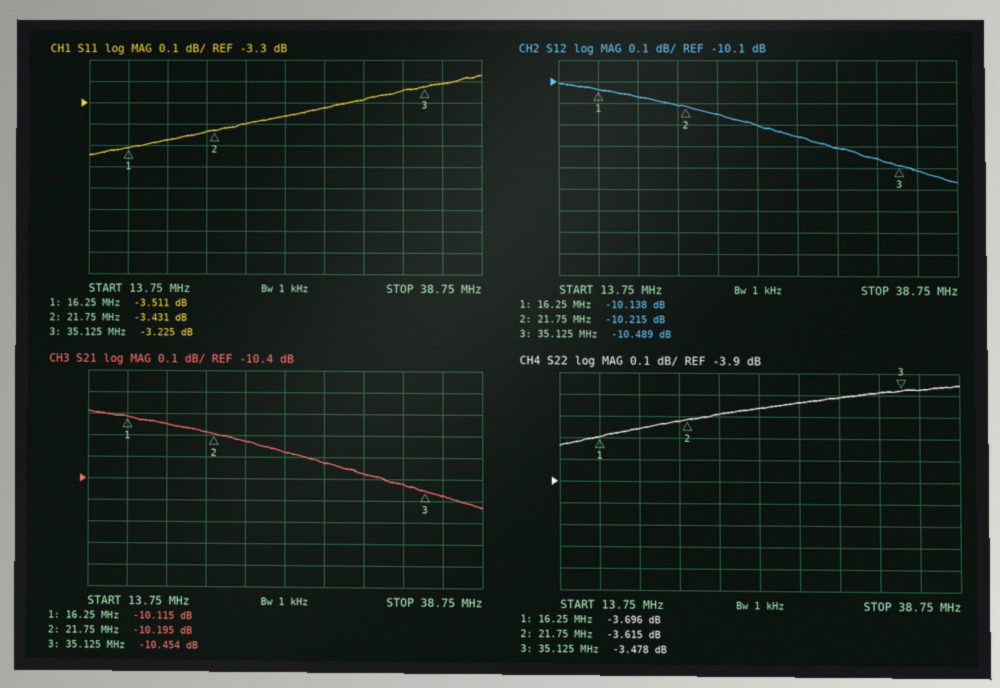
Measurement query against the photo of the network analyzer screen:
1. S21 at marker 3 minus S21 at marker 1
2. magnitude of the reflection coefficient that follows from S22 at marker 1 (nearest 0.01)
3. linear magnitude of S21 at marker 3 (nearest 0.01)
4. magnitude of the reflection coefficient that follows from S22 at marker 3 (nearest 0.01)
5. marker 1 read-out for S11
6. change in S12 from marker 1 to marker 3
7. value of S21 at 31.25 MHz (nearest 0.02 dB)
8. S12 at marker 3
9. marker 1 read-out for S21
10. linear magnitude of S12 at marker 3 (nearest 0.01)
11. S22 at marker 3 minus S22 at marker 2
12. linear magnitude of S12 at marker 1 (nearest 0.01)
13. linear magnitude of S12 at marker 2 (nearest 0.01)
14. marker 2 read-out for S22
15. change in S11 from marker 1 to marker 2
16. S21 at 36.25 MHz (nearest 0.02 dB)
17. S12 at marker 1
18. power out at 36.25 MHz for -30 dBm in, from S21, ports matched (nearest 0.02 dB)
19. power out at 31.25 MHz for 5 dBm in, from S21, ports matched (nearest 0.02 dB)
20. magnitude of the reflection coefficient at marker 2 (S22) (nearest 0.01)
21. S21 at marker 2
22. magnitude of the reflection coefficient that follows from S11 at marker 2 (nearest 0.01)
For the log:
-0.339 dB
0.65
0.30
0.67
-3.511 dB
-0.351 dB
-10.38 dB
-10.489 dB
-10.115 dB
0.30
0.137 dB
0.31
0.31
-3.615 dB
0.080 dB
-10.48 dB
-10.138 dB
-40.48 dBm
-5.38 dBm
0.66
-10.195 dB
0.67
